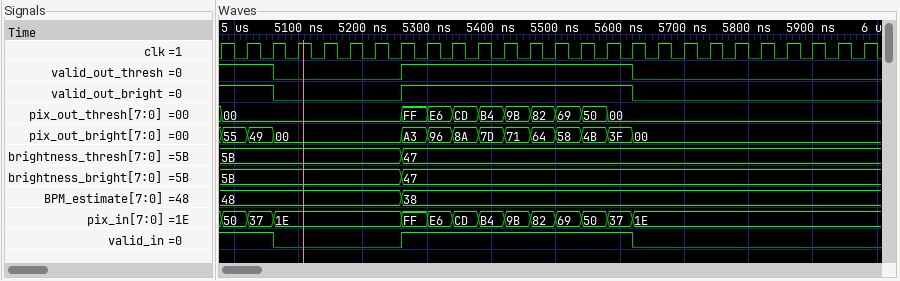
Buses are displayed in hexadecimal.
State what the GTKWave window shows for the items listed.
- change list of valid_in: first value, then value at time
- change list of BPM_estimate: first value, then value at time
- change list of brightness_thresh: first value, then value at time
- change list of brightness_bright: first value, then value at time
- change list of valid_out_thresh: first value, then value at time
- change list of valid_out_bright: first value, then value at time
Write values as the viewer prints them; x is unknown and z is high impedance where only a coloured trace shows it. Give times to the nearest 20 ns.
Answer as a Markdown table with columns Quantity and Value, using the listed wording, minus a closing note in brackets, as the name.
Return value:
| Quantity | Value |
|---|---|
| change list of valid_in: first value, then value at time | 1, 0 at 5060 ns, 1 at 5260 ns, 0 at 5620 ns |
| change list of BPM_estimate: first value, then value at time | 48, 38 at 5260 ns |
| change list of brightness_thresh: first value, then value at time | 5B, 47 at 5260 ns |
| change list of brightness_bright: first value, then value at time | 5B, 47 at 5260 ns |
| change list of valid_out_thresh: first value, then value at time | 1, 0 at 5060 ns, 1 at 5260 ns, 0 at 5620 ns |
| change list of valid_out_bright: first value, then value at time | 1, 0 at 5060 ns, 1 at 5260 ns, 0 at 5620 ns |
